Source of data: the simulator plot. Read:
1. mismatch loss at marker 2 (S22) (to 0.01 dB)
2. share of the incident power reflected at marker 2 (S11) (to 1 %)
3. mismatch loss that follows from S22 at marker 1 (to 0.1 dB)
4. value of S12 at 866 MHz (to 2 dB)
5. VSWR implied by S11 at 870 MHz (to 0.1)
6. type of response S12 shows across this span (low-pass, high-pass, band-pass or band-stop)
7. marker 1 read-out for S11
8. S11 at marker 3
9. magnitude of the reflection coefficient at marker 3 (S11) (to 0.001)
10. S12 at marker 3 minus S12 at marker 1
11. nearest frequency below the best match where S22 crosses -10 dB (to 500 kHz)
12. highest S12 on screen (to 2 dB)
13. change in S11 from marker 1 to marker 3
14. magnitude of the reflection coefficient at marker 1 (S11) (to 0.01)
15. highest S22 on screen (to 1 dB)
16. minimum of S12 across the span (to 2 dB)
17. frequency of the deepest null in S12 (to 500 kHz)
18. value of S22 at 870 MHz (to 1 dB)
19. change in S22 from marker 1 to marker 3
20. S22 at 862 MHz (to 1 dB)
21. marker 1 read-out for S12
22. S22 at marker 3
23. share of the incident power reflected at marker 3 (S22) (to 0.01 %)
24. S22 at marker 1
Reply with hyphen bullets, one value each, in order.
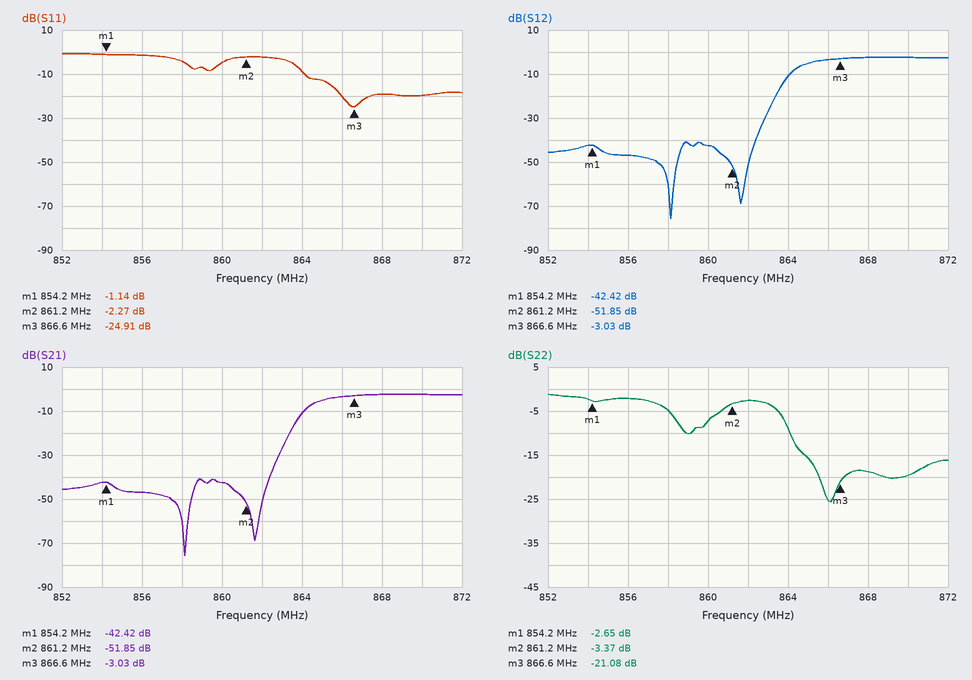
- 2.68 dB
- 59 %
- 3.4 dB
- -4 dB
- 1.2
- high-pass
- -1.14 dB
- -24.91 dB
- 0.057
- 39.39 dB
- 864.0 MHz
- -2 dB
- -23.77 dB
- 0.88
- -1 dB
- -76 dB
- 858.0 MHz
- -20 dB
- -18.43 dB
- -3 dB
- -42.42 dB
- -21.08 dB
- 0.78 %
- -2.65 dB
